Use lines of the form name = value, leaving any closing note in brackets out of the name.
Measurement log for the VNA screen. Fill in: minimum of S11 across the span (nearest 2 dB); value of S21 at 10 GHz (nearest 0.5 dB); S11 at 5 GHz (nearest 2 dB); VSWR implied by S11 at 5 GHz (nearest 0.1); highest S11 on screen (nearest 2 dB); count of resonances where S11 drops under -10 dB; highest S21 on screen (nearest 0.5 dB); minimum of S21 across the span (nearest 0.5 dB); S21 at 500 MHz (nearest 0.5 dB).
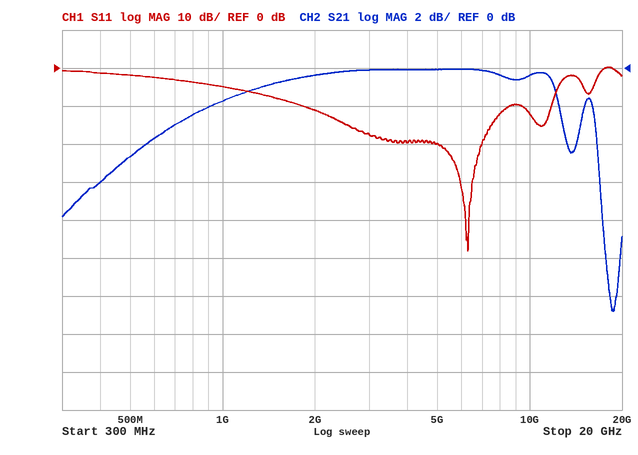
minimum of S11 across the span = -48 dB
value of S21 at 10 GHz = -0.5 dB
S11 at 5 GHz = -20 dB
VSWR implied by S11 at 5 GHz = 1.2
highest S11 on screen = 0 dB
count of resonances where S11 drops under -10 dB = 2
highest S21 on screen = 0.0 dB
minimum of S21 across the span = -13.0 dB
S21 at 500 MHz = -4.5 dB
